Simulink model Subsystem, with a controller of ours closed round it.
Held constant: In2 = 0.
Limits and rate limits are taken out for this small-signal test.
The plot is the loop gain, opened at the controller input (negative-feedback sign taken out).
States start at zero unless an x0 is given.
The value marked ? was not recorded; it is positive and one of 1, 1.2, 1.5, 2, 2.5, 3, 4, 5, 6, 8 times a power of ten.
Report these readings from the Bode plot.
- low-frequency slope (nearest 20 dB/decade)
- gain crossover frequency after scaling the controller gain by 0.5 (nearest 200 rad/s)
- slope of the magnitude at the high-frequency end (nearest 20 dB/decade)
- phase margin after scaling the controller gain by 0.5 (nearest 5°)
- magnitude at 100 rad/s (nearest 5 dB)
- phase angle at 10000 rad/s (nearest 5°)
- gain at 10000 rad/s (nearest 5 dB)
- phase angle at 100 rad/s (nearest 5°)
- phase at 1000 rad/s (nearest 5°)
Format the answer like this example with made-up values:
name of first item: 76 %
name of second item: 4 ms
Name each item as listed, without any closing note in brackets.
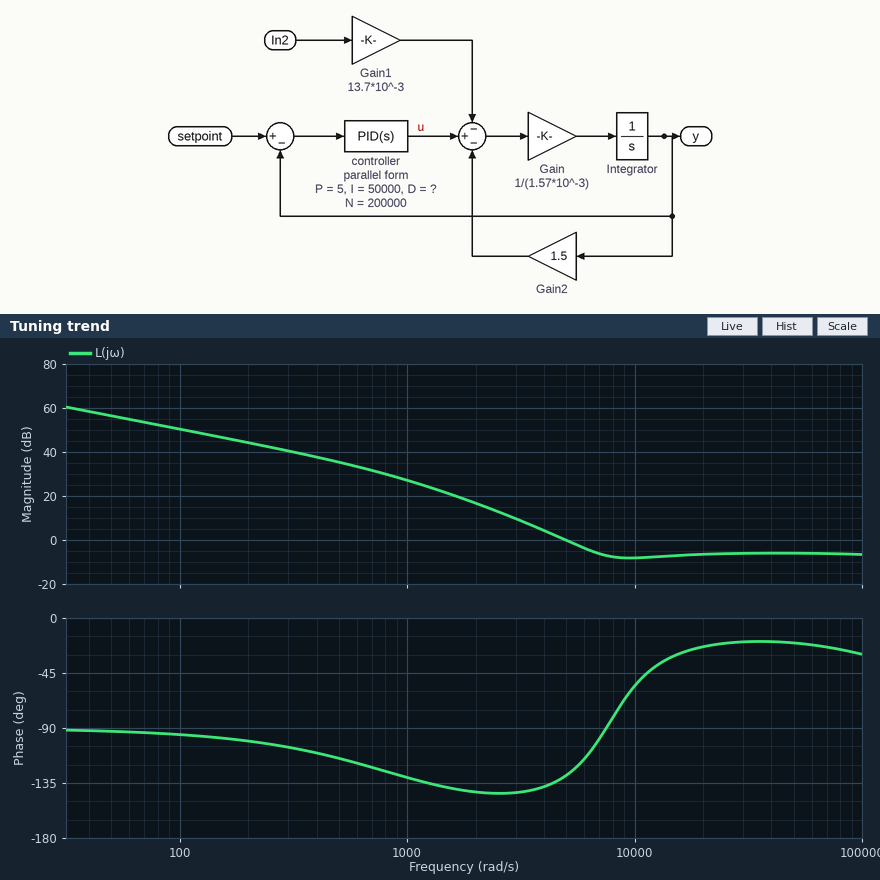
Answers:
low-frequency slope: -20 dB/decade
gain crossover frequency after scaling the controller gain by 0.5: 3600 rad/s
slope of the magnitude at the high-frequency end: 0 dB/decade
phase margin after scaling the controller gain by 0.5: 40°
magnitude at 100 rad/s: 50 dB
phase angle at 10000 rad/s: -55°
gain at 10000 rad/s: -10 dB
phase angle at 100 rad/s: -95°
phase at 1000 rad/s: -130°
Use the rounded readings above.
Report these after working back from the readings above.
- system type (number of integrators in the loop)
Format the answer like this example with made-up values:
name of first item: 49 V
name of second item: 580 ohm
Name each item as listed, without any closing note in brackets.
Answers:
system type: 1
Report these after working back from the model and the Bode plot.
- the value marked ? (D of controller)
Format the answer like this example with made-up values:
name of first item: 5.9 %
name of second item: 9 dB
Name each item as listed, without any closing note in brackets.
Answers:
the value marked ?: 0.0008
